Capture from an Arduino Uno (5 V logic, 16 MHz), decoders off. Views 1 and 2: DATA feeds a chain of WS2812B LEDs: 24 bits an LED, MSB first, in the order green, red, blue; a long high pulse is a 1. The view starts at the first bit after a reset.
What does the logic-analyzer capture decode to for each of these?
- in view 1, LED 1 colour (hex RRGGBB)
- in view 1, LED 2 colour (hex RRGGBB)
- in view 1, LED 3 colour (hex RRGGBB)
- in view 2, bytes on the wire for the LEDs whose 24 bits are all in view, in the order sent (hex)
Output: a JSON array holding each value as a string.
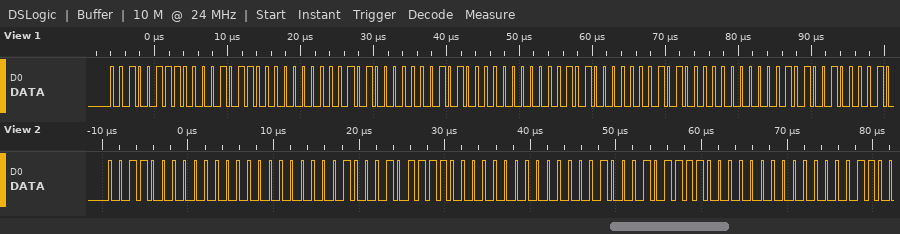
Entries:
["#0B2700", "#0A2800", "#0A2800", "30 00 02 2F 00 02 2F 00 03"]
